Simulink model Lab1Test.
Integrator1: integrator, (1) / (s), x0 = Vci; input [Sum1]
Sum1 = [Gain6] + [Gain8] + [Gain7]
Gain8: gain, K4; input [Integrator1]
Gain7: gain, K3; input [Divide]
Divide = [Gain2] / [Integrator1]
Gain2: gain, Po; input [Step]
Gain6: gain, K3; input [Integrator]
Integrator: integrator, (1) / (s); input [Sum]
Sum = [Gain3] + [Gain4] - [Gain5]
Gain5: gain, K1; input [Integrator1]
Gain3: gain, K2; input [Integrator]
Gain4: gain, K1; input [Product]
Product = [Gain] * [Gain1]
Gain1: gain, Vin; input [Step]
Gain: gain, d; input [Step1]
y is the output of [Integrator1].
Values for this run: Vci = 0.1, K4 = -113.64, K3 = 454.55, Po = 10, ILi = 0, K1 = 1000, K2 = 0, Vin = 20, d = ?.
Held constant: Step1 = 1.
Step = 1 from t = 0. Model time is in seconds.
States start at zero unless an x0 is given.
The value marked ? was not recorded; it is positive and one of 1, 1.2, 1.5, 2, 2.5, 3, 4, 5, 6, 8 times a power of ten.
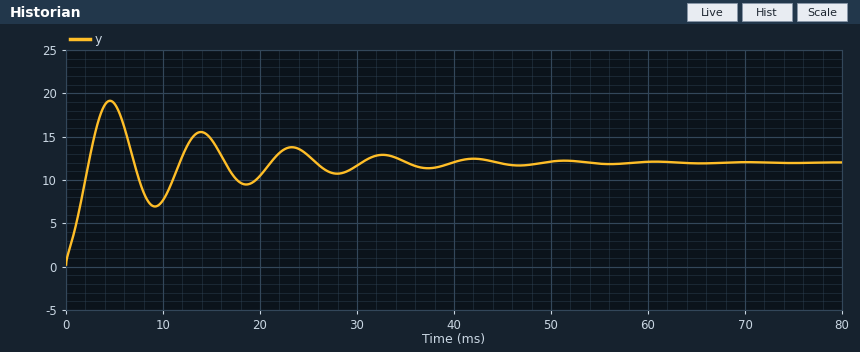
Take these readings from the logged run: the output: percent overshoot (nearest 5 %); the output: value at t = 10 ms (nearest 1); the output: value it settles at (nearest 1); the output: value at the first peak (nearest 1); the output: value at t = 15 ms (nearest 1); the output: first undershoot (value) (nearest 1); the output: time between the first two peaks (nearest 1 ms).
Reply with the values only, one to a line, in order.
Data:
60 %
8
12
19
15
7
9 ms
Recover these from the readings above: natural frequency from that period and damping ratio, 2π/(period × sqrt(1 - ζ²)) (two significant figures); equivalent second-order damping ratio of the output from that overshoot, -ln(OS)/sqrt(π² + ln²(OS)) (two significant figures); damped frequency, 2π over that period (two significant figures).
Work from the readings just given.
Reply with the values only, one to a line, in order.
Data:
0.71 rad/ms
0.16
0.70 rad/ms
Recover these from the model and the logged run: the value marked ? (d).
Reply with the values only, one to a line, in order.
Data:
0.6
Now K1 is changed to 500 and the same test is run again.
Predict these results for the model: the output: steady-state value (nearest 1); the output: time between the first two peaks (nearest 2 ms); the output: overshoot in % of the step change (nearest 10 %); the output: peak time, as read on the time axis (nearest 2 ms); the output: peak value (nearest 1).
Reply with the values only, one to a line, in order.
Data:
12
14 ms
50 %
6 ms
18
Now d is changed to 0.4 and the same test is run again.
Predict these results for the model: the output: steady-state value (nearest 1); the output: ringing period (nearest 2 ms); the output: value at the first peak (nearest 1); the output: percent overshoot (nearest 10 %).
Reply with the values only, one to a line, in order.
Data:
8
10 ms
12
50 %
